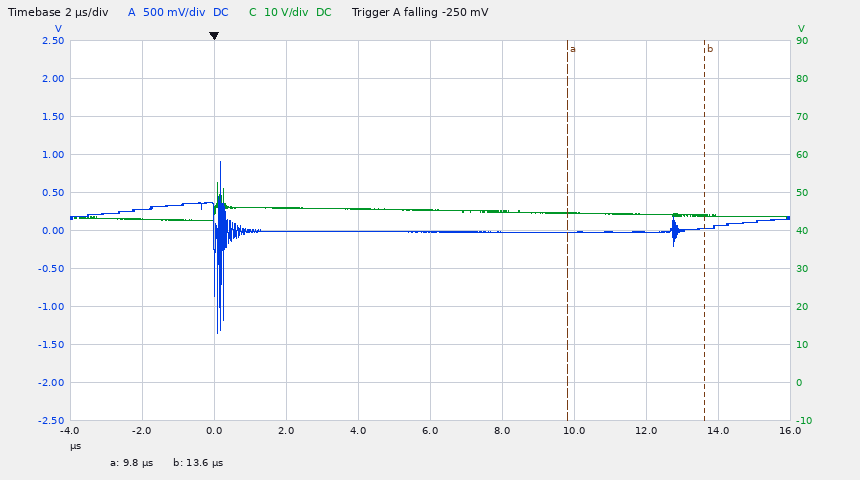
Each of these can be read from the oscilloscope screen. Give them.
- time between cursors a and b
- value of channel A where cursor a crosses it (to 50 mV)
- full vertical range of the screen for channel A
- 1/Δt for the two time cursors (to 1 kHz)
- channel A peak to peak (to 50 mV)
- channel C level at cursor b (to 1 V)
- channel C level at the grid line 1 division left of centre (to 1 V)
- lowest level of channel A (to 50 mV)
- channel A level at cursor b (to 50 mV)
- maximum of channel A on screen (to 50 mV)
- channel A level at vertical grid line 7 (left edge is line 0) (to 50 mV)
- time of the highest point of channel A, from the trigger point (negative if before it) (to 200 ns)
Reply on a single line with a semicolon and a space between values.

3.8 µs; -50 mV; 5 V; 263 kHz; 2.25 V; 44 V; 46 V; -1.35 V; 50 mV; 900 mV; -50 mV; +200 ns
